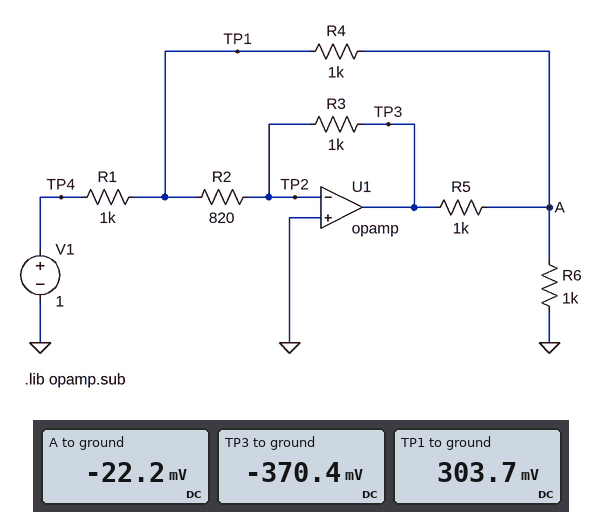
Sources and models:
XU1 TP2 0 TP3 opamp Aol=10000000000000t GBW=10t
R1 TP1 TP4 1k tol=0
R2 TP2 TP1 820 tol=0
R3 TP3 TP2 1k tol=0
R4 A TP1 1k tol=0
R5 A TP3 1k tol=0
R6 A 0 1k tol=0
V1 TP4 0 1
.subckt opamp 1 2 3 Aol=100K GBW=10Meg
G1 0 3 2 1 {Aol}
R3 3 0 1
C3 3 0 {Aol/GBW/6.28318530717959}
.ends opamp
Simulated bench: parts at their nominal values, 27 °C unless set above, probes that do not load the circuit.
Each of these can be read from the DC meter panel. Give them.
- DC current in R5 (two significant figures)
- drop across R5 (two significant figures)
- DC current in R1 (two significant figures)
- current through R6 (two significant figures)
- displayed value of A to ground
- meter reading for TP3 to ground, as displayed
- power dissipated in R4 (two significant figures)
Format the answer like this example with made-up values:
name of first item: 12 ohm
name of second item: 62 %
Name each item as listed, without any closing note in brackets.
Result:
DC current in R5: 350 µA
drop across R5: 350 mV
DC current in R1: 700 µA
current through R6: 22 µA
displayed value of A to ground: -22.2 mV
meter reading for TP3 to ground, as displayed: -370.4 mV
power dissipated in R4: 110 µW
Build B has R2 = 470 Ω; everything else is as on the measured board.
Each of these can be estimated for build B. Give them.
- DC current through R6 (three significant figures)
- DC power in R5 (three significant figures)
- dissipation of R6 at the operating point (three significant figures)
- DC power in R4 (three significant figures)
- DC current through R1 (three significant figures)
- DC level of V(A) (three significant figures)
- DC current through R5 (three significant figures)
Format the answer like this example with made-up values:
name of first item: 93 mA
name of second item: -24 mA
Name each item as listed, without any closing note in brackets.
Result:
DC current through R6: 83.5 µA
DC power in R5: 151 µW
dissipation of R6 at the operating point: 6.97 µW
DC power in R4: 93.3 µW
DC current through R1: 778 µA
DC level of V(A): -83.5 mV
DC current through R5: 389 µA
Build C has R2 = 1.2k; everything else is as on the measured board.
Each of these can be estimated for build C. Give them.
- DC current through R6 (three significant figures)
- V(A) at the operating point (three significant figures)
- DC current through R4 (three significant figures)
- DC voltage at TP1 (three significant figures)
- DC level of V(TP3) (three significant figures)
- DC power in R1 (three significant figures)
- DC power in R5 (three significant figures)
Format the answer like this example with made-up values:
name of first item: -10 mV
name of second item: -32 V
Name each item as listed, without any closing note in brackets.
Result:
DC current through R6: 20.0 µA
V(A) at the operating point: 20.0 mV
DC current through R4: 340 µA
DC voltage at TP1: 360 mV
DC level of V(TP3): -300 mV
DC power in R1: 410 µW
DC power in R5: 102 µW
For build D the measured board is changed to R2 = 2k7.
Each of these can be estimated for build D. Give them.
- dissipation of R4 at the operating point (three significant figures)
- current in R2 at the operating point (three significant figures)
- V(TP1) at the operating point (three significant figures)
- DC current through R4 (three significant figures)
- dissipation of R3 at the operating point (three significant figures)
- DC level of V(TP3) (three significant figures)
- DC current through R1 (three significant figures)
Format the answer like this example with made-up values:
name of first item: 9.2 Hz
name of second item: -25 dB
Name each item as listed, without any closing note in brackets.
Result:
dissipation of R4 at the operating point: 134 µW
current in R2 at the operating point: 171 µA
V(TP1) at the operating point: 463 mV
DC current through R4: 366 µA
dissipation of R3 at the operating point: 29.4 µW
DC level of V(TP3): -171 mV
DC current through R1: 537 µA
